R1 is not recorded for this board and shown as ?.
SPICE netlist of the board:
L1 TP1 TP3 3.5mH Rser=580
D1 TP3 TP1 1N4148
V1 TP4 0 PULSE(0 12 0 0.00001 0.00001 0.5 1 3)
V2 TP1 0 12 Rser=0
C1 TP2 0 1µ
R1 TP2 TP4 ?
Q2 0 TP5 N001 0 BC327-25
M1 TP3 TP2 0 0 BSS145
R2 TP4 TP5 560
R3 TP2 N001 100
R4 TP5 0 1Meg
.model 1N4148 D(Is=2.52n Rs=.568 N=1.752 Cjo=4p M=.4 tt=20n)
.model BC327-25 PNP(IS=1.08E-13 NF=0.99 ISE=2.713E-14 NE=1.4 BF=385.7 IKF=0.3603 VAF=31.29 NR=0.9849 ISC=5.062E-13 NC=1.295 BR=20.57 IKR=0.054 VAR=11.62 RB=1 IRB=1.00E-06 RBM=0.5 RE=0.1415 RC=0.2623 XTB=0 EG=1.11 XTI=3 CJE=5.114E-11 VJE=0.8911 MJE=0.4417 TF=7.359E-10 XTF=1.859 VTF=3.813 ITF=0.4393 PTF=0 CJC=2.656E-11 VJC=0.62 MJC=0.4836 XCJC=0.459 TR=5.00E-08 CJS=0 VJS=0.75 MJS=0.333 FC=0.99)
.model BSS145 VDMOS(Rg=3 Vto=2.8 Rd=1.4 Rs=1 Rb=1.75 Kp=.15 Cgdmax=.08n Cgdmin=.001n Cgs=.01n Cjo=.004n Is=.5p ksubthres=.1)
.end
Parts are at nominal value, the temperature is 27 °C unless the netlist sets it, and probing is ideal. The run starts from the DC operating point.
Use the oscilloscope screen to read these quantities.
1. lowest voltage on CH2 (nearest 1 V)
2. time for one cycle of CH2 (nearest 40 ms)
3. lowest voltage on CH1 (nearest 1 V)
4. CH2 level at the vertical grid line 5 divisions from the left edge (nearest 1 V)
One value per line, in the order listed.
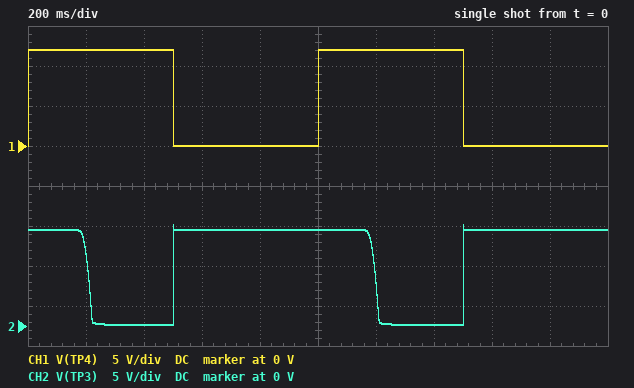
0 V
1.00 s
0 V
12 V
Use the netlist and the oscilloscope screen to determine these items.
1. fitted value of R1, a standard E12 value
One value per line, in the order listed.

680 kΩ
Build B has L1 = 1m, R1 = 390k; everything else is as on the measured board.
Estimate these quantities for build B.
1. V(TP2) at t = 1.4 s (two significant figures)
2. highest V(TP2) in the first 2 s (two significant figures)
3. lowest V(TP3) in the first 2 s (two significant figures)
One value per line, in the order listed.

7.7 V
8.7 V
73 mV
